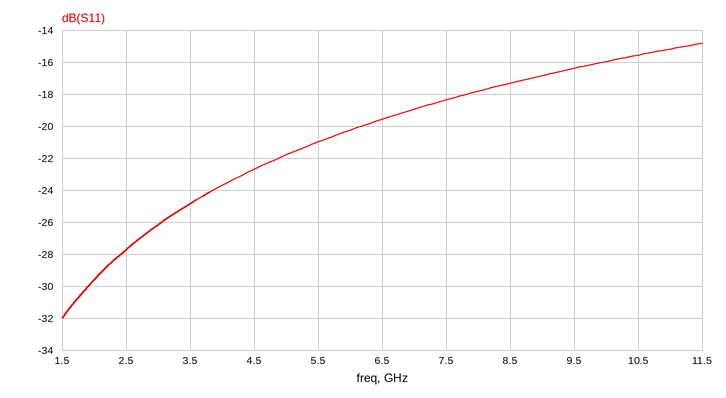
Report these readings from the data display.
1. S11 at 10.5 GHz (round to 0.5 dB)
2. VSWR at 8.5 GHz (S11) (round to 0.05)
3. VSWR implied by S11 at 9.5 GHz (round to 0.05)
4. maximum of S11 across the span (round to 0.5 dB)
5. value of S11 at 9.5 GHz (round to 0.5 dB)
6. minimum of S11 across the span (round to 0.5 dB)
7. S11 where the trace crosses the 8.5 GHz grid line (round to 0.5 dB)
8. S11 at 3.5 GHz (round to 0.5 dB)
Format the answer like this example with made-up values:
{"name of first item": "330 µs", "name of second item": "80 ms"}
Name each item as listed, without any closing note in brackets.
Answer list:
{"S11 at 10.5 GHz": "-15.5 dB", "VSWR at 8.5 GHz (S11)": "1.30", "VSWR implied by S11 at 9.5 GHz": "1.35", "maximum of S11 across the span": "-15.0 dB", "value of S11 at 9.5 GHz": "-16.5 dB", "minimum of S11 across the span": "-32.0 dB", "S11 where the trace crosses the 8.5 GHz grid line": "-17.5 dB", "S11 at 3.5 GHz": "-25.0 dB"}
